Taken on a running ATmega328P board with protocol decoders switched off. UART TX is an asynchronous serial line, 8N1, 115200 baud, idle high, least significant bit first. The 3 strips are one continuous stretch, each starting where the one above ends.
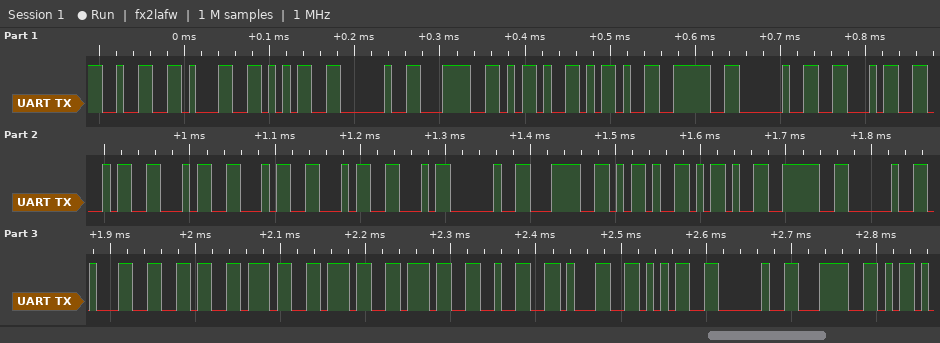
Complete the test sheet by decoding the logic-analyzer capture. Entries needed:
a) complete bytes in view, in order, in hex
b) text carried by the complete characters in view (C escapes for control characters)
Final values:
32 31 35 20 3C 2D 2D 3E 20 46 46 46 46 46 46 20 3C 2D 2D 3E 20 31 36 37 37 37 32 31 35 20 3C
"215 <--> FFFFFF <--> 16777215 <"
